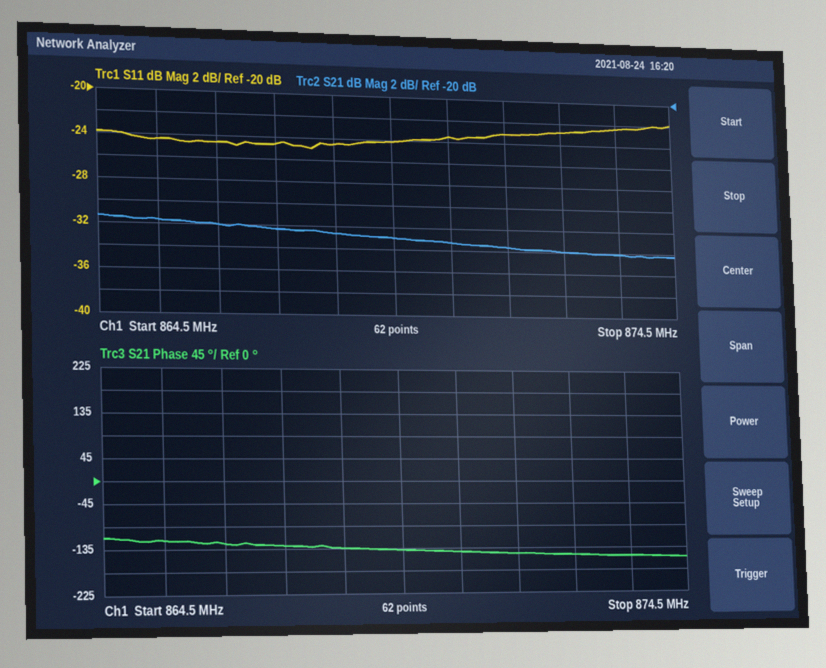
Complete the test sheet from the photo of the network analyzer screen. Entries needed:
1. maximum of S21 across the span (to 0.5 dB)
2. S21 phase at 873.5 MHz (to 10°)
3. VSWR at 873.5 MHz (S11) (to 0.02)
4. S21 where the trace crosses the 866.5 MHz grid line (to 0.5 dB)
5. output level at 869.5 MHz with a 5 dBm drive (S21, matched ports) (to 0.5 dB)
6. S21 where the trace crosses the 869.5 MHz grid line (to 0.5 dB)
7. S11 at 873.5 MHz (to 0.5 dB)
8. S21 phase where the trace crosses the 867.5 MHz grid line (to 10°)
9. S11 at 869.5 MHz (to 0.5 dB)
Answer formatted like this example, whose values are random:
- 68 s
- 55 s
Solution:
- -31.5 dB
- -150°
- 1.16
- -32.0 dB
- -28.0 dBm
- -33.0 dB
- -22.5 dB
- -130°
- -24.0 dB
